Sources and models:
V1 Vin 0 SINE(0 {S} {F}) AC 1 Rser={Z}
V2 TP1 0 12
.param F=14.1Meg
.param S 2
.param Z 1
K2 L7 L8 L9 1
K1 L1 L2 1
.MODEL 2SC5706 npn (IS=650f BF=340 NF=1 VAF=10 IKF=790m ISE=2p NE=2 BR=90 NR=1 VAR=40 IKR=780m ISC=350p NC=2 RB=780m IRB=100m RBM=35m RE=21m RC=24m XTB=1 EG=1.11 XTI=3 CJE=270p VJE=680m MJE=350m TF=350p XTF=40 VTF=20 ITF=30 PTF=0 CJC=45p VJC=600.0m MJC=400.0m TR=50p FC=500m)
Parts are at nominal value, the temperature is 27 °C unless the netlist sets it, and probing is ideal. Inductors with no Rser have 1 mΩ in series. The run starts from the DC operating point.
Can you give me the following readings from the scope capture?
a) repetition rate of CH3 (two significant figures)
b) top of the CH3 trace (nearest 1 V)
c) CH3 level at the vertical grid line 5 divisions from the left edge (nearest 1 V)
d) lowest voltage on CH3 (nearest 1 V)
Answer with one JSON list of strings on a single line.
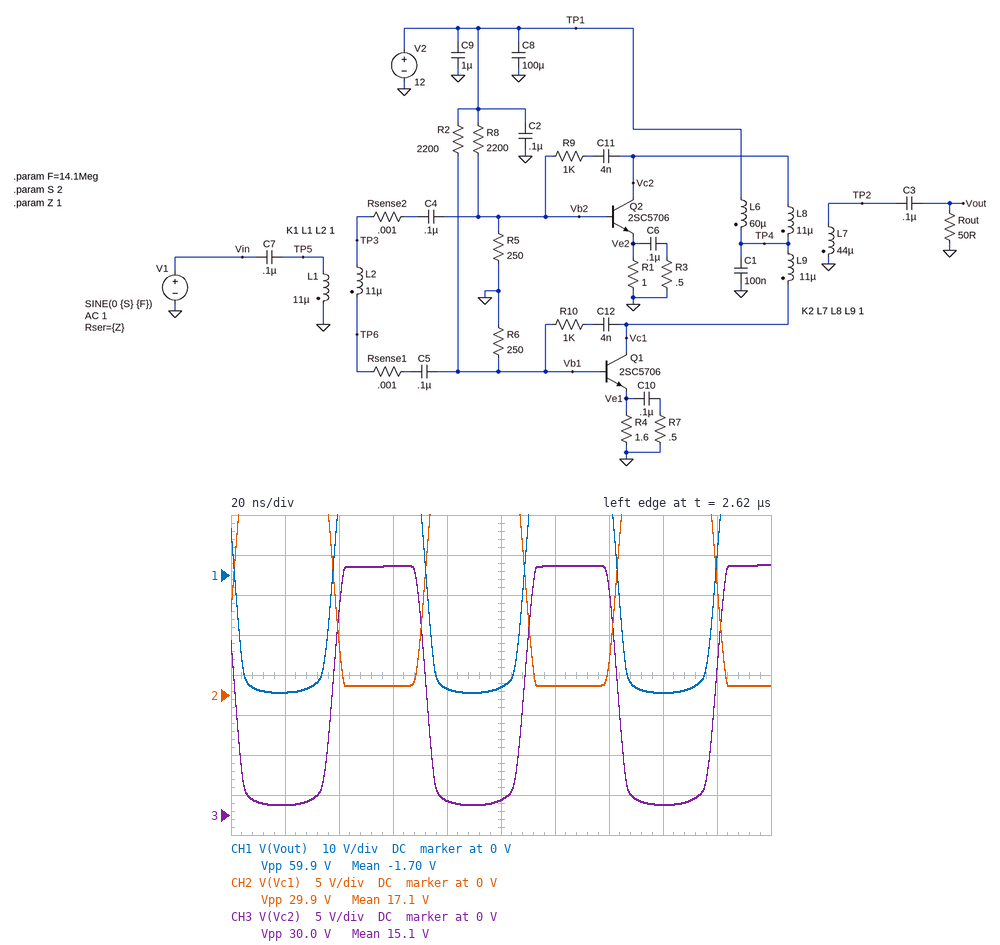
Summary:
["14 MHz", "31 V", "2 V", "1 V"]
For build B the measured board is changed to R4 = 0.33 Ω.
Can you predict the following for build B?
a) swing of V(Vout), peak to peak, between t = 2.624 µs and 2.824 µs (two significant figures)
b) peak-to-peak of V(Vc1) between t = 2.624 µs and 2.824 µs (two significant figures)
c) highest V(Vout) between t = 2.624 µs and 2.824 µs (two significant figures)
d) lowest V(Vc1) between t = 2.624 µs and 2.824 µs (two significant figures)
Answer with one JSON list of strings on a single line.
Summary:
["62 V", "31 V", "29 V", "1.3 V"]
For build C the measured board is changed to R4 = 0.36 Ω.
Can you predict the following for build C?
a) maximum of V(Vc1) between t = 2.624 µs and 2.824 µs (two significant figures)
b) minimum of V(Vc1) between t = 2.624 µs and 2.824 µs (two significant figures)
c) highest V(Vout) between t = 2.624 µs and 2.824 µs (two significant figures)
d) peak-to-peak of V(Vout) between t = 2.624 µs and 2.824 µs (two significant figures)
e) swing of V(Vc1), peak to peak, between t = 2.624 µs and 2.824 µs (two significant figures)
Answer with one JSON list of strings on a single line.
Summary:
["32 V", "1.2 V", "30 V", "62 V", "31 V"]
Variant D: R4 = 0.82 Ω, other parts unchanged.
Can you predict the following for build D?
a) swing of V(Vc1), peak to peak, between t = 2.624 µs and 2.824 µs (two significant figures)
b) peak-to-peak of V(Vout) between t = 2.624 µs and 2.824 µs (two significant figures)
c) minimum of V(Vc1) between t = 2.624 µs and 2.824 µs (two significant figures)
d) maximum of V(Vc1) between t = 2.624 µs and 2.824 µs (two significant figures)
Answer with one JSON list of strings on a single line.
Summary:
["31 V", "62 V", "950 mV", "32 V"]
